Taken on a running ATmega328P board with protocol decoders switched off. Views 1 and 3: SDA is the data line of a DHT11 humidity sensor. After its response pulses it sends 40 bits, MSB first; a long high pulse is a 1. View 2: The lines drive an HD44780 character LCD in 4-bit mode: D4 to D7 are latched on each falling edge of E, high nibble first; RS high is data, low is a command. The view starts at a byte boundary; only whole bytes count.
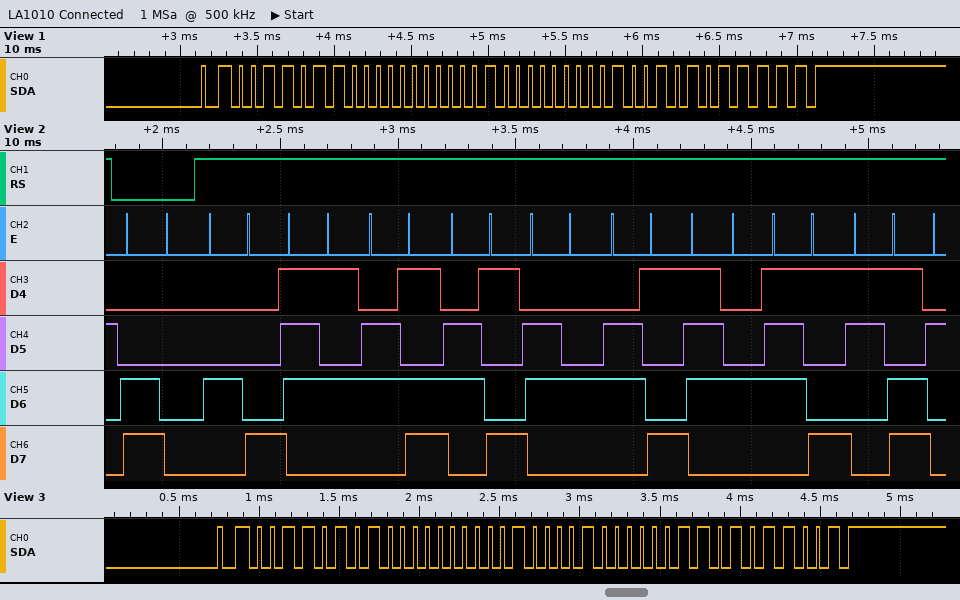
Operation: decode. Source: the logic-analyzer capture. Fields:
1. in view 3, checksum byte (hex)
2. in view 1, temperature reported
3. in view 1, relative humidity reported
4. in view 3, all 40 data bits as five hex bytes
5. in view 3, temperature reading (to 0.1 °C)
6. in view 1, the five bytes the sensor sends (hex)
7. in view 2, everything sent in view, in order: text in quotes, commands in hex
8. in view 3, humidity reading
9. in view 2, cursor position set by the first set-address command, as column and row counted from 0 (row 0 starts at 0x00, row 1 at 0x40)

0x59
32.9 °C
54 %
35 00 21 03 59
33.3 °C
36 00 20 09 5F
0xC0 "Humidity="
53 %
column 0, row 1
